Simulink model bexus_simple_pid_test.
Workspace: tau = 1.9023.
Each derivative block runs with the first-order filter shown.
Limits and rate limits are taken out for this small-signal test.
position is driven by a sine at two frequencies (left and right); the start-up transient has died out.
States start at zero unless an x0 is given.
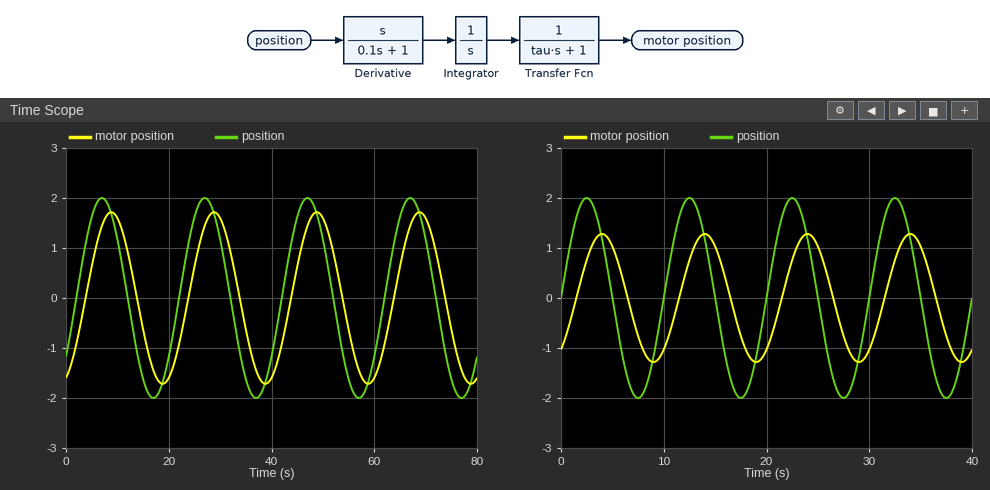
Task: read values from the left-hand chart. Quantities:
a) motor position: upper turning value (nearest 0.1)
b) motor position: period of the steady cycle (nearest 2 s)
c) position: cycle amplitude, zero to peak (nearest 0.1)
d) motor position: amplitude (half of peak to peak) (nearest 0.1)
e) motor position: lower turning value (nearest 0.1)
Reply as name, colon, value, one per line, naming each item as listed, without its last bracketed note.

motor position: upper turning value: 1.7
motor position: period of the steady cycle: 20 s
position: cycle amplitude, zero to peak: 2.0
motor position: amplitude (half of peak to peak): 1.7
motor position: lower turning value: -1.7
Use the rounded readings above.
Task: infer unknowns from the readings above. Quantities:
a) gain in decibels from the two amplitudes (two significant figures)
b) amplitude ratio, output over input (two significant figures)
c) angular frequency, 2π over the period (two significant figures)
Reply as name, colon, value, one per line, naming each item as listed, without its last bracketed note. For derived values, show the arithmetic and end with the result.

gain in decibels from the two amplitudes: 20 log10(1.7 / 2) = -1.4 dB
amplitude ratio, output over input: 1.7 / 2 = 0.85
angular frequency, 2π over the period: 2π / 20 = 0.31 rad/s
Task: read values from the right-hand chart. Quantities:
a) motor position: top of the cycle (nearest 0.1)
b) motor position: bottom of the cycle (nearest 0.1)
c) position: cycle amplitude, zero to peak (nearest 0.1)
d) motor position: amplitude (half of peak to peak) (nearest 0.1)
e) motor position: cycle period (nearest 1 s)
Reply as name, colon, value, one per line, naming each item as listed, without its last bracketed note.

motor position: top of the cycle: 1.3
motor position: bottom of the cycle: -1.3
position: cycle amplitude, zero to peak: 2.0
motor position: amplitude (half of peak to peak): 1.3
motor position: cycle period: 10 s
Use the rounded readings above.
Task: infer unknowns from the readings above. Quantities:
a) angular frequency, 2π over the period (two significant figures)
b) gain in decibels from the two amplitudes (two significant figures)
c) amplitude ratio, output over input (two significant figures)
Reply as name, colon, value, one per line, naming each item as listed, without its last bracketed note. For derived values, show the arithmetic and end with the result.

angular frequency, 2π over the period: 2π / 10 = 0.63 rad/s
gain in decibels from the two amplitudes: 20 log10(1.3 / 2) = -3.7 dB
amplitude ratio, output over input: 1.3 / 2 = 0.65
